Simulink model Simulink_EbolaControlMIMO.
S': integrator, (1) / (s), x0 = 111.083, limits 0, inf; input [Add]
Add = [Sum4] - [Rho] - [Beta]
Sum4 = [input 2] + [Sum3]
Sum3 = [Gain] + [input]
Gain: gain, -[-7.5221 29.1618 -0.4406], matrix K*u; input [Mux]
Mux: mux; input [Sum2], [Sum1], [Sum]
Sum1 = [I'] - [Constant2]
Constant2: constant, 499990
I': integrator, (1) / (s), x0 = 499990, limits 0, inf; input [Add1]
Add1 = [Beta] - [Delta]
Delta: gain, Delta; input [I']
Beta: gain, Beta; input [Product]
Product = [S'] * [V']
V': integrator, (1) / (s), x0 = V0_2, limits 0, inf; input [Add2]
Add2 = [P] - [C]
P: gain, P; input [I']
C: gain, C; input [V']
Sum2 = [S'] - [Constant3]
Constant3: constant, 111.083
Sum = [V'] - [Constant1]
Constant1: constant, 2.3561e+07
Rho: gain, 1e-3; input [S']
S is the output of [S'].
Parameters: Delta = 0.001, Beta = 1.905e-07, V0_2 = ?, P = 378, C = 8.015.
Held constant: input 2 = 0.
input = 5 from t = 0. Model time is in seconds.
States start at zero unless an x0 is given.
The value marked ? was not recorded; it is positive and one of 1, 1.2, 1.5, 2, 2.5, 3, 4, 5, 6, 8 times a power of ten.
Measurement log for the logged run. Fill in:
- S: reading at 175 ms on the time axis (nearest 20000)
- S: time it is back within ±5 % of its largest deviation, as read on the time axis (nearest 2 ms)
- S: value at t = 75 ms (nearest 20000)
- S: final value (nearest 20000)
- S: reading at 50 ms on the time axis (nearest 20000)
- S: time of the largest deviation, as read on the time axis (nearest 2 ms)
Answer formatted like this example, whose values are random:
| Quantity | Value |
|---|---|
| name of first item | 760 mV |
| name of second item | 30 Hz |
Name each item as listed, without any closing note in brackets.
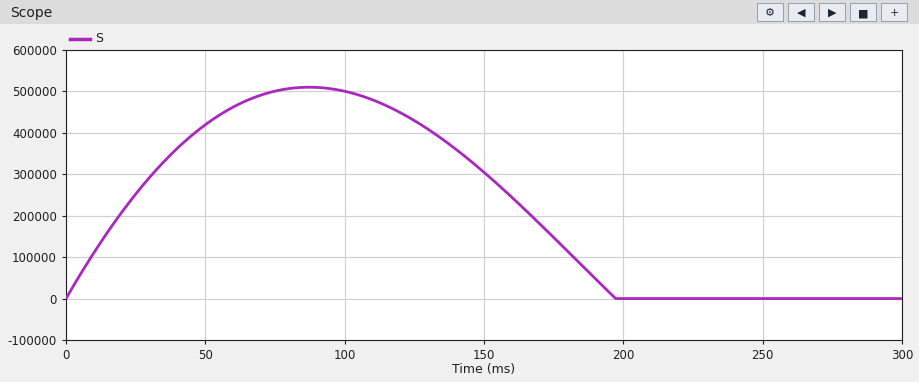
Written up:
| Quantity | Value |
|---|---|
| S: reading at 175 ms on the time axis | 140000 |
| S: time it is back within ±5 % of its largest deviation, as read on the time axis | 194 ms |
| S: value at t = 75 ms | 500000 |
| S: final value | 0 |
| S: reading at 50 ms on the time axis | 420000 |
| S: time of the largest deviation, as read on the time axis | 88 ms |
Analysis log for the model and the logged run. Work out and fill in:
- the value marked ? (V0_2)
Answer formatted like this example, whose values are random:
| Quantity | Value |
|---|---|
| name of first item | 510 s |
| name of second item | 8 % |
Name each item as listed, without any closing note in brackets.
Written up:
| Quantity | Value |
|---|---|
| the value marked ? | 5e+07 |
